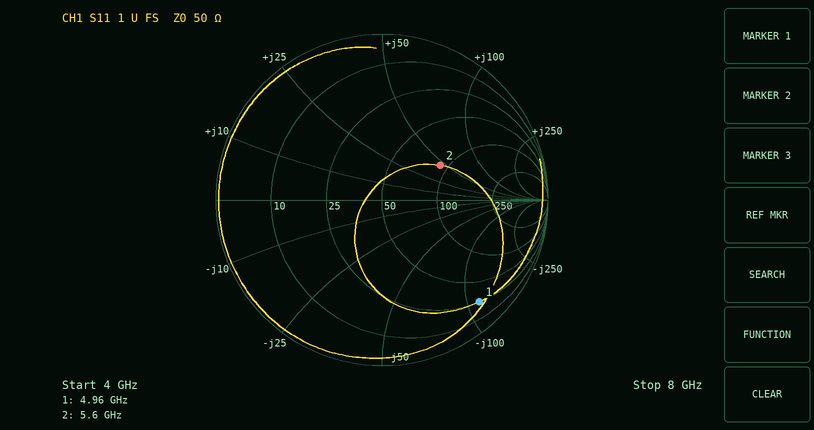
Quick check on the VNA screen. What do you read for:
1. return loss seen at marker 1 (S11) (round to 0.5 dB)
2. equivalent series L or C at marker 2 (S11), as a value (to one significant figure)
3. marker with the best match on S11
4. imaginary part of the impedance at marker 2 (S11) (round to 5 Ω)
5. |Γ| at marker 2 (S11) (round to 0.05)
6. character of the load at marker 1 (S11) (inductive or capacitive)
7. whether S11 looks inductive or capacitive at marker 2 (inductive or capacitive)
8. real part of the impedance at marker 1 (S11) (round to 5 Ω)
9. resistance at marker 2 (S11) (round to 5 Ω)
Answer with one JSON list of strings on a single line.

["1.5 dB", "1 nH", "marker 2", "+45 Ω", "0.40", "capacitive", "inductive", "25 Ω", "90 Ω"]
